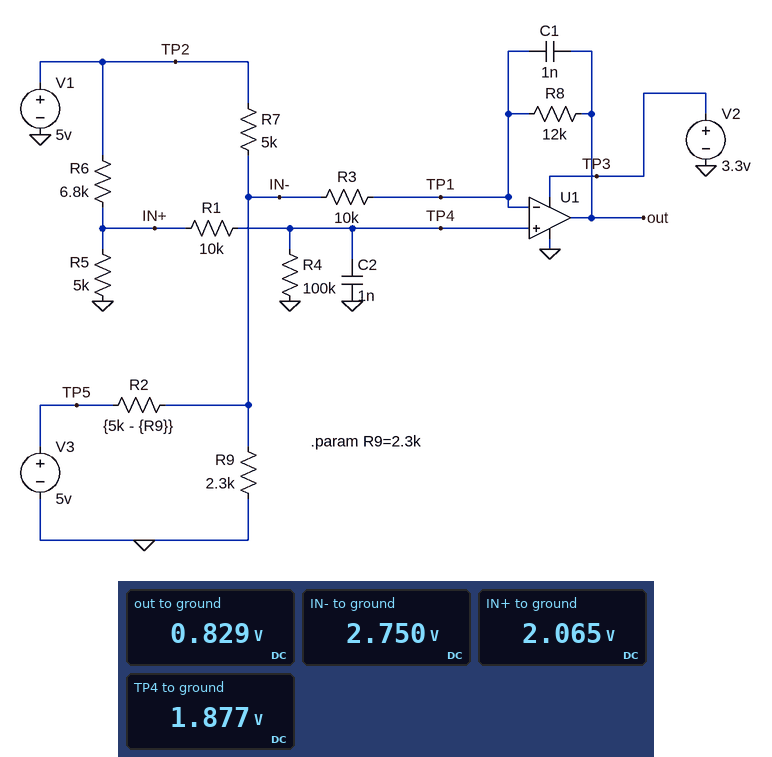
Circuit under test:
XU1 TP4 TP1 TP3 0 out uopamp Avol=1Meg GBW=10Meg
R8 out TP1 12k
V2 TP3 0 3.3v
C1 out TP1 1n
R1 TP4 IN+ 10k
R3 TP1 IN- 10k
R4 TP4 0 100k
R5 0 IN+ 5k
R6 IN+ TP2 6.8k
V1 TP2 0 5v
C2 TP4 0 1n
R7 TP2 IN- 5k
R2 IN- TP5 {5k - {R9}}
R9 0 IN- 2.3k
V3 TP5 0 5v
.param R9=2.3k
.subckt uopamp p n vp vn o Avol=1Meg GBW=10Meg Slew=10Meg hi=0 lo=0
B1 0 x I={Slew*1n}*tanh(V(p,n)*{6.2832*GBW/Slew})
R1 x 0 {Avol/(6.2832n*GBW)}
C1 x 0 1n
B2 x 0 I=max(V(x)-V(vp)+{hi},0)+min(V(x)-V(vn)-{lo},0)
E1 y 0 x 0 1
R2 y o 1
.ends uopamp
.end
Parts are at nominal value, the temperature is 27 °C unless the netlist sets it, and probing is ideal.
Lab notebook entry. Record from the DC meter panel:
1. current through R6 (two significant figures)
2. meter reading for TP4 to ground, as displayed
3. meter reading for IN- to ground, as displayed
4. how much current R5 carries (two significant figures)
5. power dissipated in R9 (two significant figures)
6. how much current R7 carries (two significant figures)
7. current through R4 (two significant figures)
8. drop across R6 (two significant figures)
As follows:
430 µA
1.877 V
2.750 V
410 µA
3.3 mW
450 µA
19 µA
2.9 V
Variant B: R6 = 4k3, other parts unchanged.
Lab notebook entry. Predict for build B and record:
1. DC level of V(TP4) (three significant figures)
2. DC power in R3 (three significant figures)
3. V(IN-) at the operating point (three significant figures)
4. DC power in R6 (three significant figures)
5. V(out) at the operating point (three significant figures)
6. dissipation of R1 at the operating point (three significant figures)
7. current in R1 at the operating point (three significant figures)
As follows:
2.39 V
16.3 µW
2.80 V
1.30 mW
1.91 V
5.73 µW
23.9 µA
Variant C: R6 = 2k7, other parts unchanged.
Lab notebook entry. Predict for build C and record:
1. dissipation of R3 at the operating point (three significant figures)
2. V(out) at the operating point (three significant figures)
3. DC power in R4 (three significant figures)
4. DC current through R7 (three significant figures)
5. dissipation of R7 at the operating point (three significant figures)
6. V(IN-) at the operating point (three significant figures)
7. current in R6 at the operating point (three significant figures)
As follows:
383 nW
2.98 V
84.4 µW
431 µA
930 µW
2.84 V
668 µA
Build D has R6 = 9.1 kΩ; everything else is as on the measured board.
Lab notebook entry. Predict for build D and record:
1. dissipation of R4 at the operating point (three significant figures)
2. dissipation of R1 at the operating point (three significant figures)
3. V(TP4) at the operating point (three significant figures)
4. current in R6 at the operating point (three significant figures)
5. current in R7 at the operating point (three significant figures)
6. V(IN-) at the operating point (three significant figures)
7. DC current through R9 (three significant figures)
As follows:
24.5 µW
2.45 µW
1.57 V
360 µA
456 µA
2.72 V
1.18 mA
